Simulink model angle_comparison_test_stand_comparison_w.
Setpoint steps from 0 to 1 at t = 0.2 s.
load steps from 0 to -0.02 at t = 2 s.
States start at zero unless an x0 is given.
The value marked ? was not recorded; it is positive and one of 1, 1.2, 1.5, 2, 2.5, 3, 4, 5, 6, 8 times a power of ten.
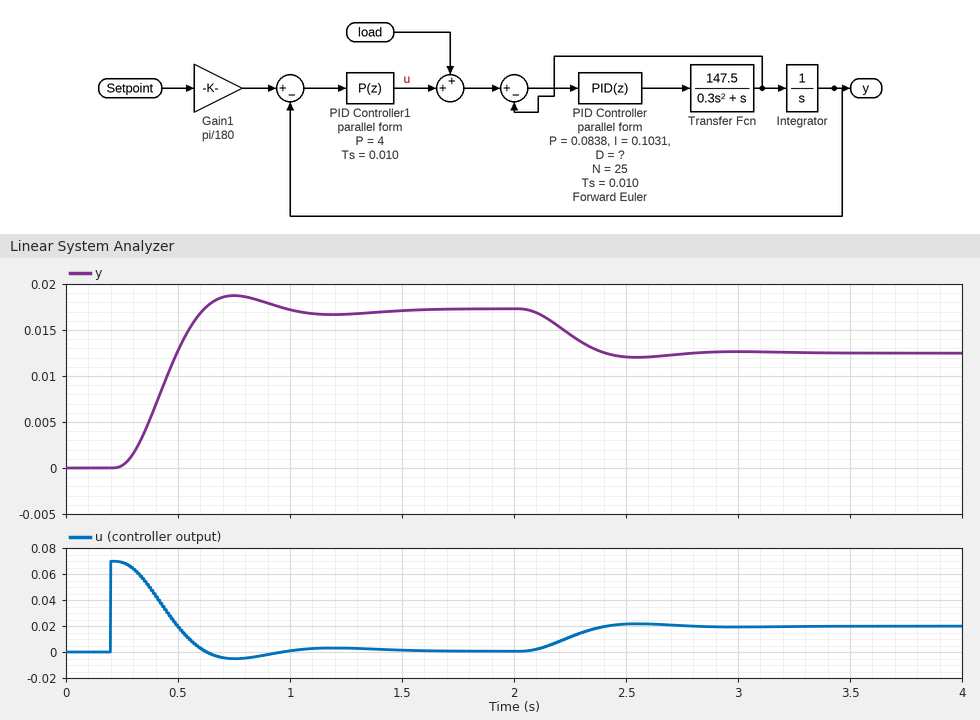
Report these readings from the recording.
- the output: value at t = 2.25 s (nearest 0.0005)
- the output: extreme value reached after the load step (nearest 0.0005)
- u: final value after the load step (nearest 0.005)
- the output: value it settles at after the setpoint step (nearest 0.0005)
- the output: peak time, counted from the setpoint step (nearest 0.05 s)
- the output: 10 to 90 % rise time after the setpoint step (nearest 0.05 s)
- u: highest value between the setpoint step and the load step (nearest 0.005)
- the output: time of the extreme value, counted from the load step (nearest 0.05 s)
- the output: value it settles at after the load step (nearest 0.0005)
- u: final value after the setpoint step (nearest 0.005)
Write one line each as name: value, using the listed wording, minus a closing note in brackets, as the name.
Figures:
the output: value at t = 2.25 s: 0.0145
the output: extreme value reached after the load step: 0.0120
u: final value after the load step: 0.020
the output: value it settles at after the setpoint step: 0.0175
the output: peak time, counted from the setpoint step: 0.55 s
the output: 10 to 90 % rise time after the setpoint step: 0.25 s
u: highest value between the setpoint step and the load step: 0.070
the output: time of the extreme value, counted from the load step: 0.55 s
the output: value it settles at after the load step: 0.0125
u: final value after the setpoint step: 0.000
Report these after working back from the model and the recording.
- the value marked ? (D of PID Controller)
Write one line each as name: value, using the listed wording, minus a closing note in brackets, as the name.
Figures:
the value marked ?: 0.015
